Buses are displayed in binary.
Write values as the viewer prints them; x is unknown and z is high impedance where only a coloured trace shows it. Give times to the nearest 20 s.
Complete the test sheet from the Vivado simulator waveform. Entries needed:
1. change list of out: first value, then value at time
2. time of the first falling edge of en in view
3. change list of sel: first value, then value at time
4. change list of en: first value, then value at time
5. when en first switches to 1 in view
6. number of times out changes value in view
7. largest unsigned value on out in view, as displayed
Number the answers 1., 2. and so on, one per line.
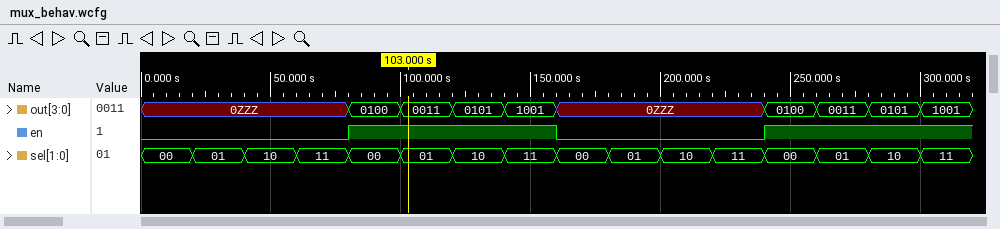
1. 0ZZZ, 0100 at 80 s, 0011 at 100 s, 0101 at 120 s, 1001 at 140 s, 0ZZZ at 160 s, 0100 at 240 s, 0011 at 260 s, 0101 at 280 s, 1001 at 300 s
2. 160 s
3. 00, 01 at 20 s, 10 at 40 s, 11 at 60 s, 00 at 80 s, 01 at 100 s, 10 at 120 s, 11 at 140 s, 00 at 160 s, 01 at 180 s, 10 at 200 s, 11 at 220 s, 00 at 240 s, 01 at 260 s, 10 at 280 s, 11 at 300 s
4. 0, 1 at 80 s, 0 at 160 s, 1 at 240 s
5. 80 s
6. 9
7. 1001
